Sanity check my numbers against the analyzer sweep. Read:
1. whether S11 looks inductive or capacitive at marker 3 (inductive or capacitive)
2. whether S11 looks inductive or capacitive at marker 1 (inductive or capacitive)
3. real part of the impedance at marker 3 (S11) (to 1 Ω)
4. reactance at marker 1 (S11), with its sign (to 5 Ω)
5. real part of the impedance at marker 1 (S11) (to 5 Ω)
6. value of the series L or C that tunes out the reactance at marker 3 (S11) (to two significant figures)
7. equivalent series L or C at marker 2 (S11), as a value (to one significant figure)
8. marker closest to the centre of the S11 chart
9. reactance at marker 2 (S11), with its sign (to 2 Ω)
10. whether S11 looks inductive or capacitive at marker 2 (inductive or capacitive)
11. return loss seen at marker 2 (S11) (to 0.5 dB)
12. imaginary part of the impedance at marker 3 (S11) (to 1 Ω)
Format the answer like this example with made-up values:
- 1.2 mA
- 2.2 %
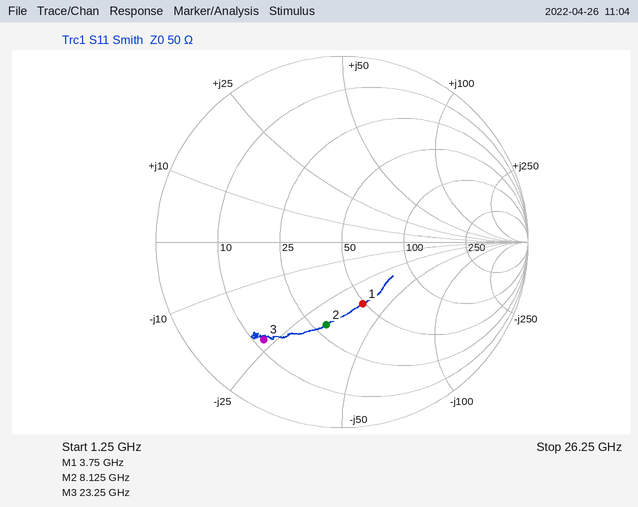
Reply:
- capacitive
- capacitive
- 12 Ω
- -35 Ω
- 50 Ω
- 160 pH
- 600 fF
- marker 1
- -32 Ω
- capacitive
- 7.0 dB
- -23 Ω
